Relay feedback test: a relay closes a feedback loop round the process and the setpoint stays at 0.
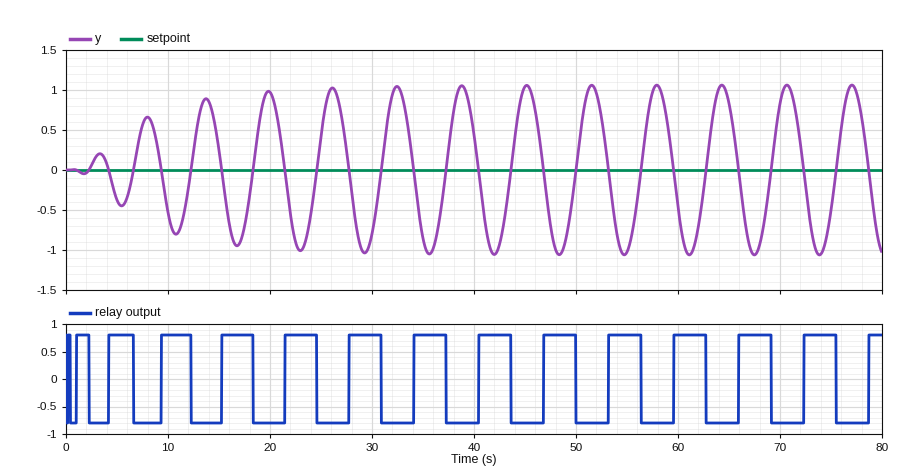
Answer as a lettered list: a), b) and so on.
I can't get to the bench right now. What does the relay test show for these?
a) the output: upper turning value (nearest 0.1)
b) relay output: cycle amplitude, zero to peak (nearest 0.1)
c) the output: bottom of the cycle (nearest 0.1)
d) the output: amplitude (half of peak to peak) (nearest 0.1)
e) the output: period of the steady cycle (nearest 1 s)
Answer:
a) 1.1
b) 0.8
c) -1.1
d) 1.1
e) 6 s
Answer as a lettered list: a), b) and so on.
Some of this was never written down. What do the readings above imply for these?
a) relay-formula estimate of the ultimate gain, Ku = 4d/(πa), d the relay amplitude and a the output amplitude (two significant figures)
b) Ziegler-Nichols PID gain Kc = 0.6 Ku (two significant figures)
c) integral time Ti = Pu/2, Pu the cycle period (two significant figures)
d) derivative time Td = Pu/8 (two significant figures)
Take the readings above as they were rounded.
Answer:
a) 0.93
b) 0.56
c) 3.0 s
d) 0.75 s
